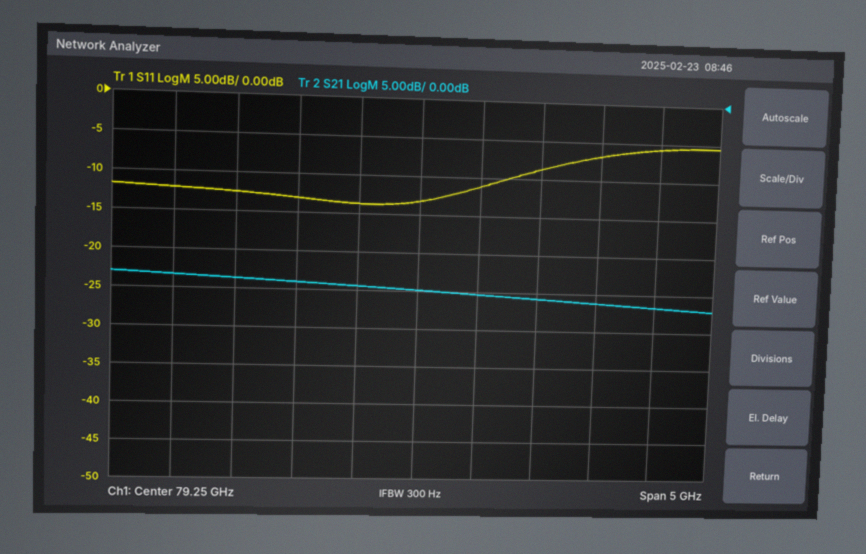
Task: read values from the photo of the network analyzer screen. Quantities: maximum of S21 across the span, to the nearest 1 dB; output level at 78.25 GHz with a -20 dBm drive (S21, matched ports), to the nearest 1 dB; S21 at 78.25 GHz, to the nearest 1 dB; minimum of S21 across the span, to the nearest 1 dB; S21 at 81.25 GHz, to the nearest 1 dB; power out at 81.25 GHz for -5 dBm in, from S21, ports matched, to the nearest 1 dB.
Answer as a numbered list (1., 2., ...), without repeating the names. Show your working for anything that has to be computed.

1. -23 dB
2. -20 dBm + (-24 dB) = -44 dBm
3. -24 dB
4. -27 dB
5. -27 dB
6. -5 dBm + (-27 dB) = -32 dBm
